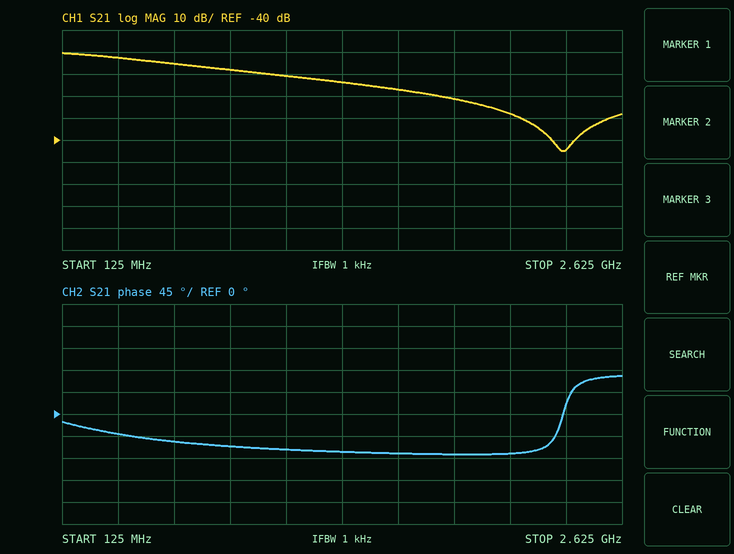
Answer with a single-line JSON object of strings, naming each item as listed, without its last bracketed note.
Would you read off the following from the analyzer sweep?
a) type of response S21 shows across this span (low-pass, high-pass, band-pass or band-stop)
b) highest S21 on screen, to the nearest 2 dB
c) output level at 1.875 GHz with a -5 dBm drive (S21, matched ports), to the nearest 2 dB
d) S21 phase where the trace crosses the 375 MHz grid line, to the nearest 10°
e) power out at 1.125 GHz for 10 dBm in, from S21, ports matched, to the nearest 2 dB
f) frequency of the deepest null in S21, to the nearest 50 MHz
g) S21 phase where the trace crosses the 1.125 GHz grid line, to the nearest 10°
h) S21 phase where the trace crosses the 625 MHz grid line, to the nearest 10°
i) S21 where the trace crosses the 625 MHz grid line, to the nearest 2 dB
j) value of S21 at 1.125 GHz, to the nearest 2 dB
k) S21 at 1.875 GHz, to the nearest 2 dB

{"type of response S21 shows across this span": "low-pass", "highest S21 on screen, to the nearest 2 dB": "0 dB", "output level at 1.875 GHz with a -5 dBm drive (S21, matched ports), to the nearest 2 dB": "-26 dBm", "S21 phase where the trace crosses the 375 MHz grid line, to the nearest 10°": "-40°", "power out at 1.125 GHz for 10 dBm in, from S21, ports matched, to the nearest 2 dB": "0 dBm", "frequency of the deepest null in S21, to the nearest 50 MHz": "2.35 GHz", "S21 phase where the trace crosses the 1.125 GHz grid line, to the nearest 10°": "-70°", "S21 phase where the trace crosses the 625 MHz grid line, to the nearest 10°": "-60°", "S21 where the trace crosses the 625 MHz grid line, to the nearest 2 dB": "-6 dB", "value of S21 at 1.125 GHz, to the nearest 2 dB": "-10 dB", "S21 at 1.875 GHz, to the nearest 2 dB": "-22 dB"}
